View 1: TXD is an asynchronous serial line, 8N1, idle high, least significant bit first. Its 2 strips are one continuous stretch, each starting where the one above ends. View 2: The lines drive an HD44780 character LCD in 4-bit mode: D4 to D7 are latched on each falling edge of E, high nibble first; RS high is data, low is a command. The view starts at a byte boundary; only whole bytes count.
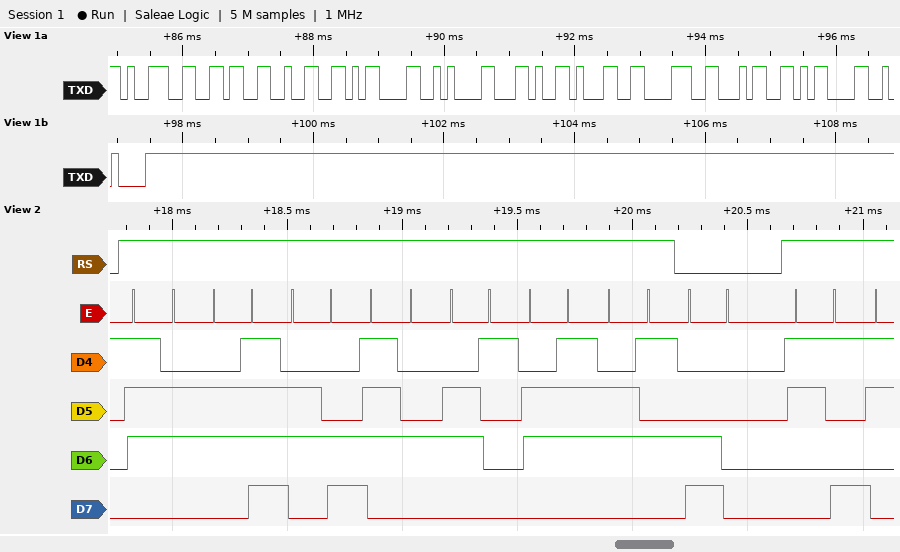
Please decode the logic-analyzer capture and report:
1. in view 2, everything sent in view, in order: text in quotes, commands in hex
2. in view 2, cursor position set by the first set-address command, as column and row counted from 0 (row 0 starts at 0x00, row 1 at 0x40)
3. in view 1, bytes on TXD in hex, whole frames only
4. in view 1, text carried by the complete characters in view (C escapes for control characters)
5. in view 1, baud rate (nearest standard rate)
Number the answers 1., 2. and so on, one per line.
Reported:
1. "voltage" 0xC0 "9"
2. column 0, row 1
3. 39 36 32 0D 0A 2C 31 38 34 0D 0A
4. "962\r\n,184\r\n"
5. 9600 baud
